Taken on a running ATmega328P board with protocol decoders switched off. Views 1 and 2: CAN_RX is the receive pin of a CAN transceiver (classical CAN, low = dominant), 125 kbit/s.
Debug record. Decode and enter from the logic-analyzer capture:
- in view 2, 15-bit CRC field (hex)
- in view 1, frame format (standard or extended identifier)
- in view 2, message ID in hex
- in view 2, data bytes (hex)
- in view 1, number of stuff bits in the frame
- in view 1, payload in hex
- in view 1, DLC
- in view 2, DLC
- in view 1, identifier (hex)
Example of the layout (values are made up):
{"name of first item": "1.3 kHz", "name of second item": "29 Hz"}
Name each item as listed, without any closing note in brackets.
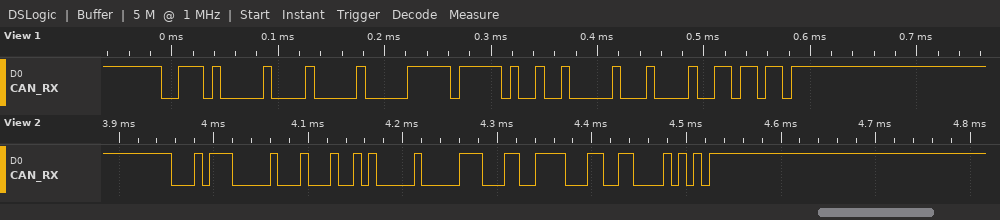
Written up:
{"in view 2, 15-bit CRC field": "0x330A", "in view 1, frame format": "standard", "in view 2, message ID in hex": "0x170", "in view 2, data bytes": "4A 00 63 3C", "in view 1, number of stuff bits in the frame": "6", "in view 1, payload in hex": "00 FF C9 00", "in view 1, DLC": "4", "in view 2, DLC": "4", "in view 1, identifier": "0x3A0"}
